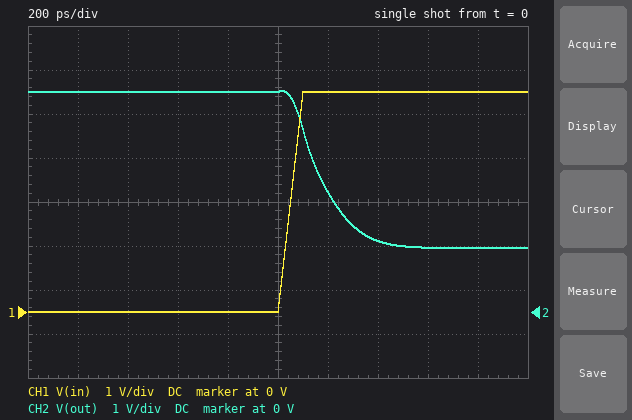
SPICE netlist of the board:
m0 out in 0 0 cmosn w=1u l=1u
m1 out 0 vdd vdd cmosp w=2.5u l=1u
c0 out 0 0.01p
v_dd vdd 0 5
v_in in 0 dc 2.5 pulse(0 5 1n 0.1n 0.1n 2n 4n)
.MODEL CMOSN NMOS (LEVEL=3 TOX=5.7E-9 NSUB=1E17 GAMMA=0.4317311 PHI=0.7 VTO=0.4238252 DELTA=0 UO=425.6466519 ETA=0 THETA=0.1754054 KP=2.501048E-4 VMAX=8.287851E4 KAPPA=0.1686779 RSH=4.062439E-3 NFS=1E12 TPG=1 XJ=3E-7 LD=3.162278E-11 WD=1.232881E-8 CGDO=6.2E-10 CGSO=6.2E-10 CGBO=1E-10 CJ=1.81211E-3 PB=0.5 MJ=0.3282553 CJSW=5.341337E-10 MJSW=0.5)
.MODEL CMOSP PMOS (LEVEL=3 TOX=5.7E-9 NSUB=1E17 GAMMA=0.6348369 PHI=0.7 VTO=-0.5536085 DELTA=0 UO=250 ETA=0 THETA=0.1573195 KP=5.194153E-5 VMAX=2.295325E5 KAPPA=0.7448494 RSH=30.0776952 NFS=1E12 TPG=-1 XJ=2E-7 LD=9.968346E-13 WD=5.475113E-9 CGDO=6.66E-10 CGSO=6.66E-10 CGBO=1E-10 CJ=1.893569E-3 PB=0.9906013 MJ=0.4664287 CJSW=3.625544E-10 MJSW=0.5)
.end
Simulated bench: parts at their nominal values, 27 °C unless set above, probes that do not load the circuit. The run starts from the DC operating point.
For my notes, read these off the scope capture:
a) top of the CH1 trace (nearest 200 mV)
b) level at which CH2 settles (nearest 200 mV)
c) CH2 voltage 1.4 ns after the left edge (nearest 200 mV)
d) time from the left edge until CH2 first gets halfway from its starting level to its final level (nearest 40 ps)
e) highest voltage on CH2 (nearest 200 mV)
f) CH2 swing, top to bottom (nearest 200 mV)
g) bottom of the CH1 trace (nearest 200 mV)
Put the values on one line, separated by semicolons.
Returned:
5.0 V; 1.4 V; 1.6 V; 1.16 ns; 5.0 V; 3.6 V; 0 V
